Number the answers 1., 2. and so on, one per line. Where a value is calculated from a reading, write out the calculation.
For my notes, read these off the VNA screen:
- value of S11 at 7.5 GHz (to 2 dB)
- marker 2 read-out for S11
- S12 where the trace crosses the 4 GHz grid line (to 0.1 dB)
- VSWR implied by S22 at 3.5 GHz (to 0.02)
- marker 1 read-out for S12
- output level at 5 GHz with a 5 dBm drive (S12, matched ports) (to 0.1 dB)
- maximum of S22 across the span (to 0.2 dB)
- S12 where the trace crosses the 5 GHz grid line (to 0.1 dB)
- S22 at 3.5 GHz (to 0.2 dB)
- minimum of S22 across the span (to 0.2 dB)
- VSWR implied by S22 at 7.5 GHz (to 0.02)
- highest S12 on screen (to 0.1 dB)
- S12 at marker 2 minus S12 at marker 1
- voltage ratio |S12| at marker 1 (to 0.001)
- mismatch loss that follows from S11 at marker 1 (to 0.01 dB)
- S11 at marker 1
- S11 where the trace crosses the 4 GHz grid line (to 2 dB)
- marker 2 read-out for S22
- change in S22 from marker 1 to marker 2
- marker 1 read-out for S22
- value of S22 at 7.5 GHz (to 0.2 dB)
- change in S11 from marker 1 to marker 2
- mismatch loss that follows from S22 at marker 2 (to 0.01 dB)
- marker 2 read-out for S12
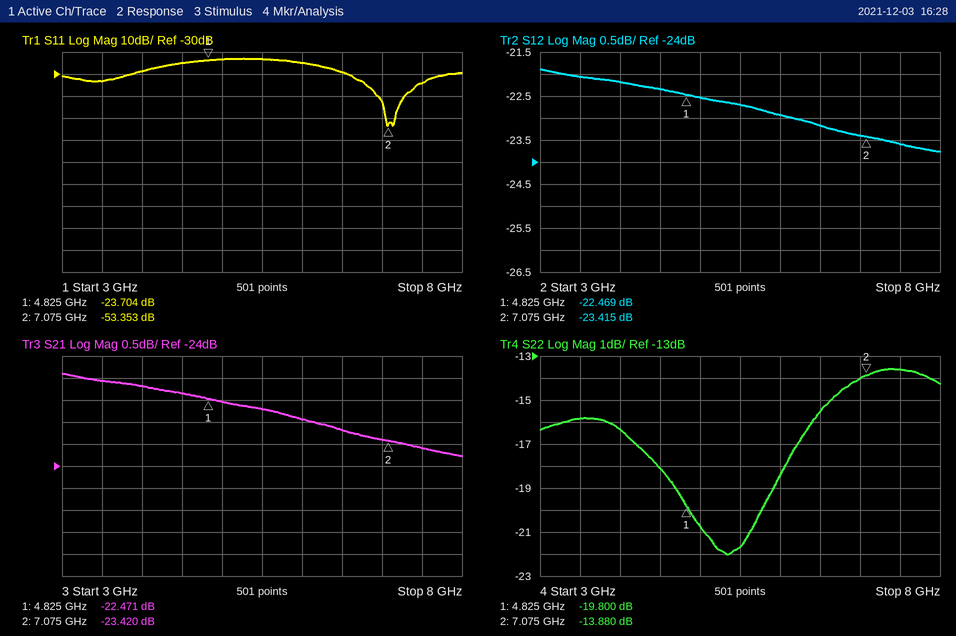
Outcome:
1. -34 dB
2. -53.353 dB
3. -22.2 dB
4. |Γ| = 10^(-15.8/20) = 0.1622; VSWR = (1 + 0.1622)/(1 − 0.1622) ≈ 1.39, so 1.38 to the nearest 0.02
5. -22.469 dB
6. 5 dBm + (-22.5 dB) = -17.5 dBm
7. -13.6 dB
8. -22.5 dB
9. -15.8 dB
10. -22.0 dB
11. |Γ| = 10^(-13.6/20) = 0.2089; VSWR = (1 + 0.2089)/(1 − 0.2089) ≈ 1.53, so 1.52 to the nearest 0.02
12. -21.9 dB
13. -23.415 − (-22.469) = -0.946 dB
14. 10^(-22.469/20) ≈ 0.075
15. −10 log10(1 − 10^(-23.704/10)) ≈ 0.02 dB
16. -23.704 dB
17. -28 dB
18. -13.880 dB
19. -13.88 − (-19.8) = 5.920 dB
20. -19.800 dB
21. -13.6 dB
22. -53.353 − (-23.704) = -29.649 dB
23. −10 log10(1 − 10^(-13.88/10)) ≈ 0.18 dB
24. -23.415 dB
